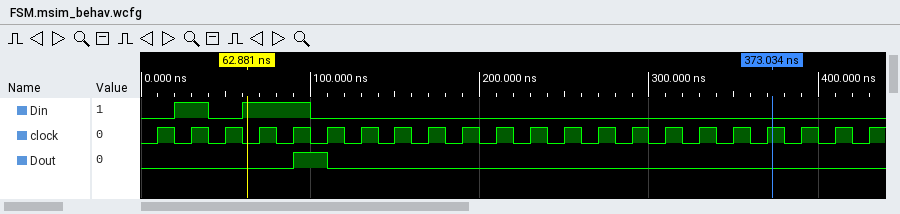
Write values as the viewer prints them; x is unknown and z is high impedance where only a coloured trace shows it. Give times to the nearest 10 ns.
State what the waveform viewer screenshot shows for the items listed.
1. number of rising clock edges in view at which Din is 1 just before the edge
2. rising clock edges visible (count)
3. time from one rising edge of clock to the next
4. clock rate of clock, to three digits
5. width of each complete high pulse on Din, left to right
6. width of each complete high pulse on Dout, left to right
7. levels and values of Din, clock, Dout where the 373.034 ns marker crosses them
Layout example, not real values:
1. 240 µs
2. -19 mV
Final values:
1. 3
2. 22
3. 20 ns
4. 50.0 MHz
5. 20 ns, 40 ns
6. 20 ns
7. Din=0, clock=1, Dout=0
